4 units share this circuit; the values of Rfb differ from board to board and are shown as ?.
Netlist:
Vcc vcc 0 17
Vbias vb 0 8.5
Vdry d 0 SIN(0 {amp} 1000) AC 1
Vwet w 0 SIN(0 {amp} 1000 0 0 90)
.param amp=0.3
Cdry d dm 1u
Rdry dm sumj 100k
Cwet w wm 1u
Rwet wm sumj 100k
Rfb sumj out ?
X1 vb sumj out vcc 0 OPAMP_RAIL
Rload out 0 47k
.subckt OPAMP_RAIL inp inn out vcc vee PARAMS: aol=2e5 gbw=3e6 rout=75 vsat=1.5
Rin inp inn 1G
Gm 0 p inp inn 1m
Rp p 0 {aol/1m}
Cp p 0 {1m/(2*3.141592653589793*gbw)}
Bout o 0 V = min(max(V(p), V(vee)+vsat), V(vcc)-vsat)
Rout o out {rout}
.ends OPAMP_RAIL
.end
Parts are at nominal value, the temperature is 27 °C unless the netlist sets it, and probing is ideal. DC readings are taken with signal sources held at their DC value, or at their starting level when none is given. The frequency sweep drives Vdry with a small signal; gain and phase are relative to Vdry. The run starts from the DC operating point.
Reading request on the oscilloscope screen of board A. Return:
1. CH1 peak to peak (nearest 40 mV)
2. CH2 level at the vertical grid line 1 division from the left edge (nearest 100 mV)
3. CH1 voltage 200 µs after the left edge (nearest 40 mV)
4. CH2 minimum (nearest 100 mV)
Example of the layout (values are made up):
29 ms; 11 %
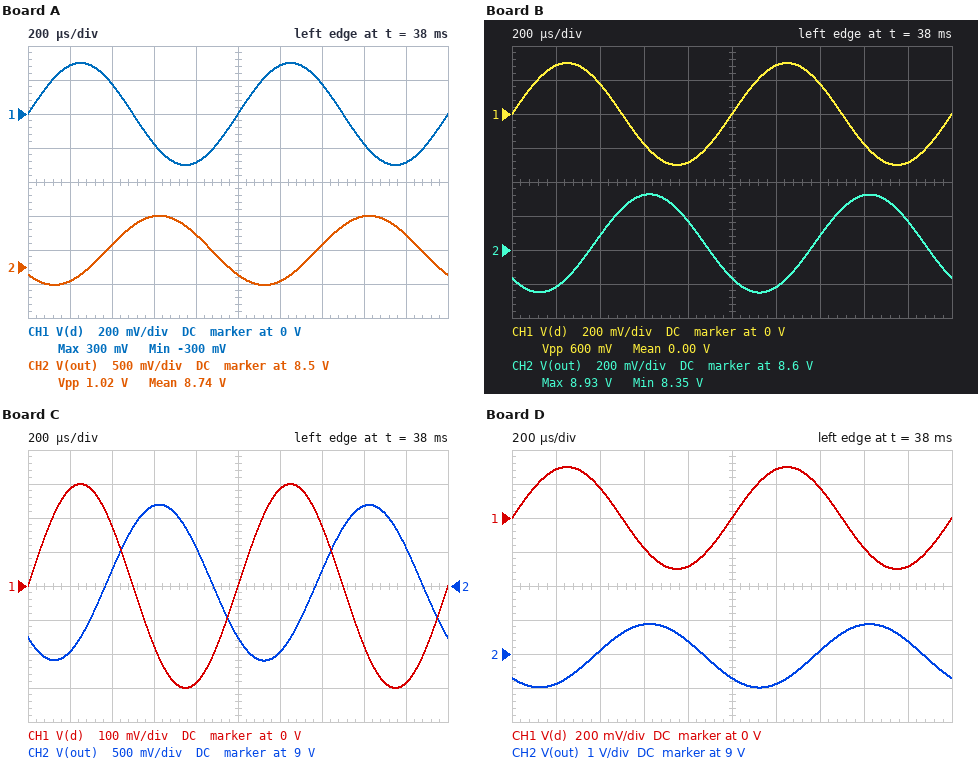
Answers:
600 mV; 8.3 V; 280 mV; 8.2 V
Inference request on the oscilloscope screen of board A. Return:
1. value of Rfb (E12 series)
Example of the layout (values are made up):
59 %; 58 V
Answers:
120 kΩ
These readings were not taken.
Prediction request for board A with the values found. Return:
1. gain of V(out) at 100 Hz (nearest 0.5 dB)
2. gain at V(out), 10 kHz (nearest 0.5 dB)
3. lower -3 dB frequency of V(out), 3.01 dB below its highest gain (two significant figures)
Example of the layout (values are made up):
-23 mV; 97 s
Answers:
1.5 dB; 1.5 dB; 1.6 Hz
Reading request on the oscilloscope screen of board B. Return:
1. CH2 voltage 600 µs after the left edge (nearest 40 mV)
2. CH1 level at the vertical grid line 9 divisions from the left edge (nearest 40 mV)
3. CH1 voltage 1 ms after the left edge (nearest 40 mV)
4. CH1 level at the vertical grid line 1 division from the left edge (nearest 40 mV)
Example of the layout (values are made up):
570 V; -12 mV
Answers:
8.92 V; -280 mV; 0 V; 280 mV
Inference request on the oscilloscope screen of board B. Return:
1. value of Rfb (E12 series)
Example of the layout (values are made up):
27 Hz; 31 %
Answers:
68 kΩ
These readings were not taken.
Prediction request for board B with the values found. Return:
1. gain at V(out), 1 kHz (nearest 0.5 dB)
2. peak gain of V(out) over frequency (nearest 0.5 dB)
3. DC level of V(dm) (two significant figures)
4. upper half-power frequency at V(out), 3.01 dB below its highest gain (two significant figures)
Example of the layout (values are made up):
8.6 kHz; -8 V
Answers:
-3.5 dB; -3.5 dB; 8.5 V; 1.3 MHz
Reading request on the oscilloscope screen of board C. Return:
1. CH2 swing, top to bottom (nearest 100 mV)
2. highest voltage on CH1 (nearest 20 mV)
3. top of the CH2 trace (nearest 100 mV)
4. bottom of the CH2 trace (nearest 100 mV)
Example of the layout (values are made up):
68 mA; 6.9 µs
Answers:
2.3 V; 300 mV; 10.2 V; 7.9 V
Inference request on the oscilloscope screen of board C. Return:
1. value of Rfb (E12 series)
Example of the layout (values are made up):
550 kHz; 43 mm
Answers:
270 kΩ
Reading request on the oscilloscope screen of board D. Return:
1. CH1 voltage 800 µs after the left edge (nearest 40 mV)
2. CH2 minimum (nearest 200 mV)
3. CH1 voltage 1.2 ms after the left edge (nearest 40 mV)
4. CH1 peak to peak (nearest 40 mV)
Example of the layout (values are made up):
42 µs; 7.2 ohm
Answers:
-280 mV; 8.0 V; 280 mV; 600 mV
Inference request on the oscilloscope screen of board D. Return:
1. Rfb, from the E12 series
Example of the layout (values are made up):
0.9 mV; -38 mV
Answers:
220 kΩ
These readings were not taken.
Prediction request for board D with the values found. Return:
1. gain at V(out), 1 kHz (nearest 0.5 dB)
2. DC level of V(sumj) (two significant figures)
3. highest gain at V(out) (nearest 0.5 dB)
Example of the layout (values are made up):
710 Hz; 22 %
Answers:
7.0 dB; 8.5 V; 7.0 dB
